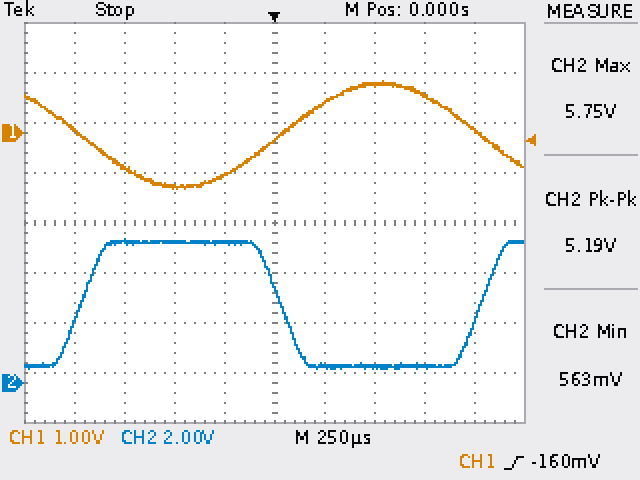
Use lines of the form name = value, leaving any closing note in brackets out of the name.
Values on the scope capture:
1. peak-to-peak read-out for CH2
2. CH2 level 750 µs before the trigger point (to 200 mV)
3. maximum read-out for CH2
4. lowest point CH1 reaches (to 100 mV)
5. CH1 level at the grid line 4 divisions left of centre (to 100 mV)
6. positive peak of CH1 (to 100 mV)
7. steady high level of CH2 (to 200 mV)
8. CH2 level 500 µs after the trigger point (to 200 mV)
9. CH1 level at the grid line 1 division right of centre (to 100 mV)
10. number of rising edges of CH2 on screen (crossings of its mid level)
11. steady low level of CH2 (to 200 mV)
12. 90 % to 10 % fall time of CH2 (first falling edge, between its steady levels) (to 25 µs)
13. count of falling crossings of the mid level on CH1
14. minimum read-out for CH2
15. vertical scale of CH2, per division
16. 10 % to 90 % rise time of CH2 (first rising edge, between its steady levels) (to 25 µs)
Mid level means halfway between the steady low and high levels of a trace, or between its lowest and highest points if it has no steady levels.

peak-to-peak read-out for CH2 = 5.19 V
CH2 level 750 µs before the trigger point = 5.6 V
maximum read-out for CH2 = 5.75 V
lowest point CH1 reaches = -1.1 V
CH1 level at the grid line 4 divisions left of centre = 100 mV
positive peak of CH1 = 1.0 V
steady high level of CH2 = 5.6 V
CH2 level 500 µs after the trigger point = 600 mV
CH1 level at the grid line 1 division right of centre = 600 mV
number of rising edges of CH2 on screen = 2
steady low level of CH2 = 600 mV
90 % to 10 % fall time of CH2 (first falling edge, between its steady levels) = 200 µs
count of falling crossings of the mid level on CH1 = 2
minimum read-out for CH2 = 563 mV
vertical scale of CH2, per division = 2 V
10 % to 90 % rise time of CH2 (first rising edge, between its steady levels) = 200 µs
